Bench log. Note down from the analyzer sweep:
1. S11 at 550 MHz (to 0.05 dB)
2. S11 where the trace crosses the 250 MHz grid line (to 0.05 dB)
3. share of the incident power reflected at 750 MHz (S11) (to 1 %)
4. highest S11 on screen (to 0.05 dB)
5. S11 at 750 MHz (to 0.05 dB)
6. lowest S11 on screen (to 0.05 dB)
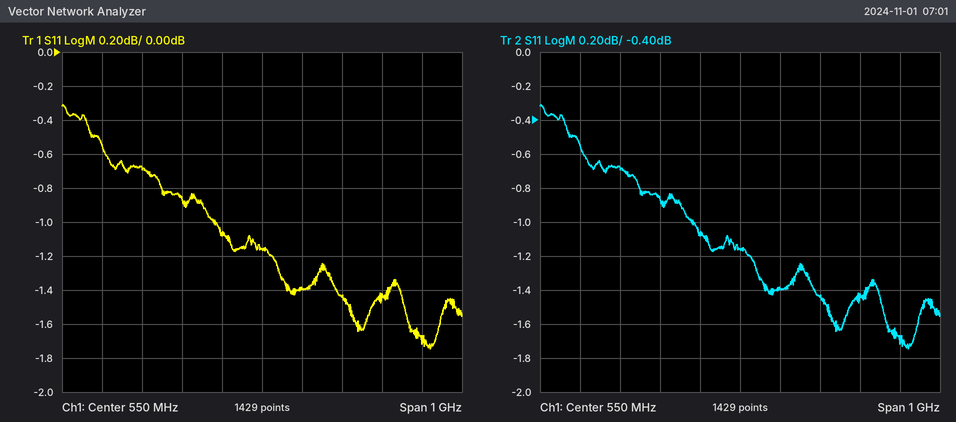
-1.15 dB
-0.70 dB
72 %
-0.30 dB
-1.45 dB
-1.75 dB
